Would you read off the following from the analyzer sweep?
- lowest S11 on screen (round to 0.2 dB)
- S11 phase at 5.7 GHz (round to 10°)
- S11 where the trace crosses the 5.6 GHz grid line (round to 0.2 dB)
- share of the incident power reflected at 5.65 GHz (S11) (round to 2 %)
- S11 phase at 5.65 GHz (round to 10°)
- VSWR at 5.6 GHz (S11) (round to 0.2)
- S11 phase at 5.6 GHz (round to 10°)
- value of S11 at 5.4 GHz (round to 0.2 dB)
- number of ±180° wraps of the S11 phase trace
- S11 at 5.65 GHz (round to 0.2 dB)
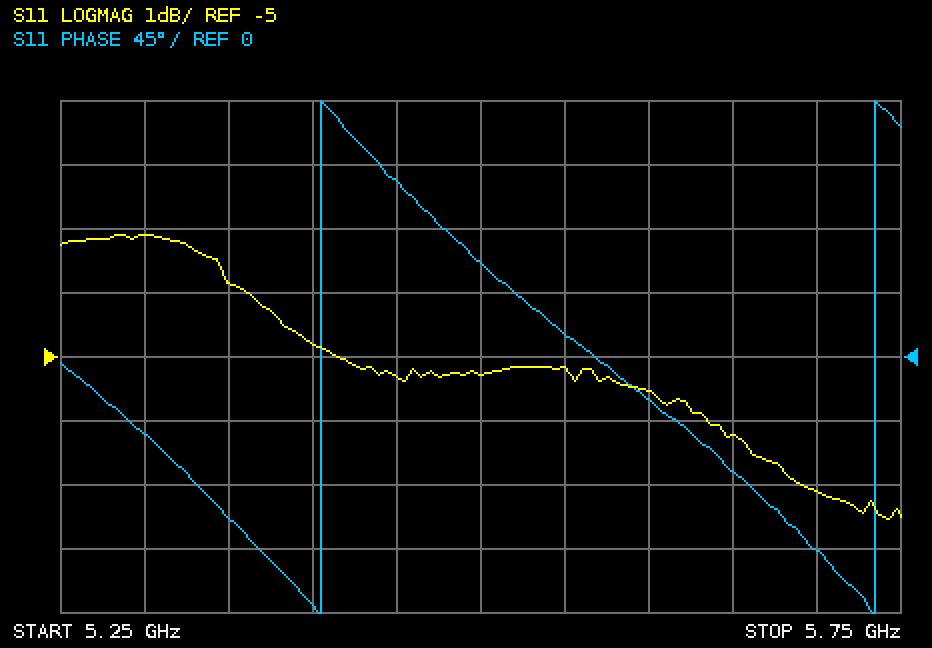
-7.6 dB
-140°
-5.6 dB
24 %
-80°
3.2
-30°
-4.8 dB
2
-6.2 dB
